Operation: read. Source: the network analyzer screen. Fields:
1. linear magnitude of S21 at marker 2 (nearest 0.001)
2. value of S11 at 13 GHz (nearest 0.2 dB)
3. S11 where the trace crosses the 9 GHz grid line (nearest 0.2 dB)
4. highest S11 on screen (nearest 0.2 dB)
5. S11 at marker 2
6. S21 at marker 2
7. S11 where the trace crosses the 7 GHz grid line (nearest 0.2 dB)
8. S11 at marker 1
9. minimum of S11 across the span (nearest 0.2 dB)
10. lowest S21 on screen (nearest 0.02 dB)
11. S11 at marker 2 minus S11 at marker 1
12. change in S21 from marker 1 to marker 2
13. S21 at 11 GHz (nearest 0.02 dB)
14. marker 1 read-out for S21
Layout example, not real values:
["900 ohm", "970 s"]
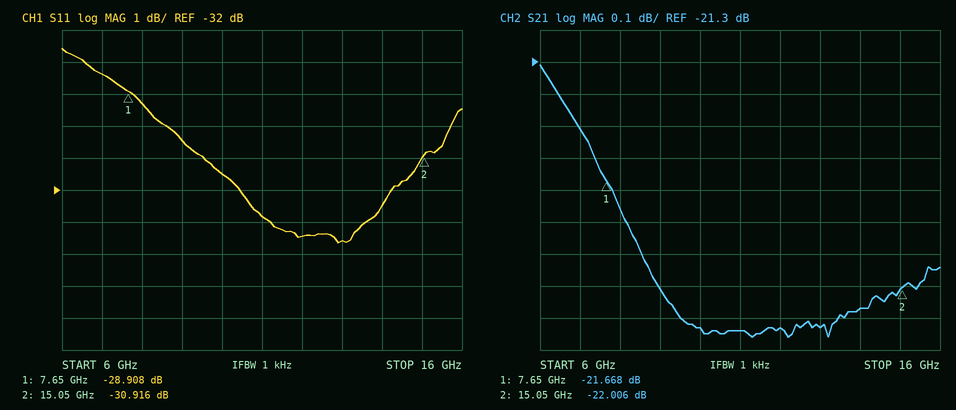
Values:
["0.079", "-33.6 dB", "-30.4 dB", "-27.6 dB", "-30.916 dB", "-22.006 dB", "-28.4 dB", "-28.908 dB", "-33.6 dB", "-22.16 dB", "-2.008 dB", "-0.338 dB", "-22.14 dB", "-21.668 dB"]
